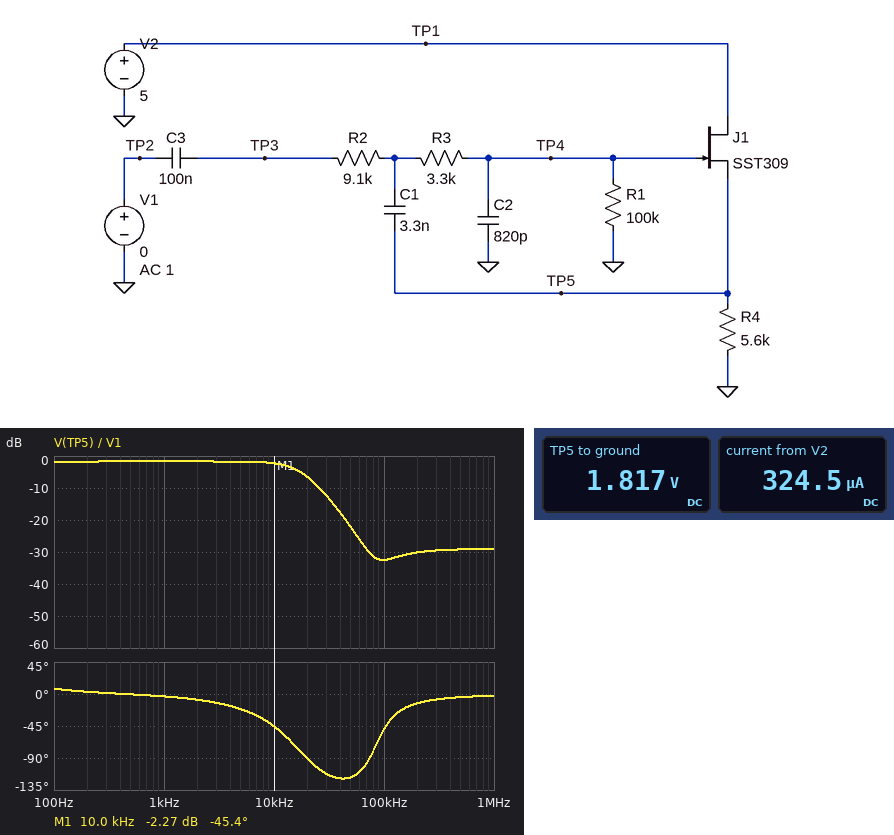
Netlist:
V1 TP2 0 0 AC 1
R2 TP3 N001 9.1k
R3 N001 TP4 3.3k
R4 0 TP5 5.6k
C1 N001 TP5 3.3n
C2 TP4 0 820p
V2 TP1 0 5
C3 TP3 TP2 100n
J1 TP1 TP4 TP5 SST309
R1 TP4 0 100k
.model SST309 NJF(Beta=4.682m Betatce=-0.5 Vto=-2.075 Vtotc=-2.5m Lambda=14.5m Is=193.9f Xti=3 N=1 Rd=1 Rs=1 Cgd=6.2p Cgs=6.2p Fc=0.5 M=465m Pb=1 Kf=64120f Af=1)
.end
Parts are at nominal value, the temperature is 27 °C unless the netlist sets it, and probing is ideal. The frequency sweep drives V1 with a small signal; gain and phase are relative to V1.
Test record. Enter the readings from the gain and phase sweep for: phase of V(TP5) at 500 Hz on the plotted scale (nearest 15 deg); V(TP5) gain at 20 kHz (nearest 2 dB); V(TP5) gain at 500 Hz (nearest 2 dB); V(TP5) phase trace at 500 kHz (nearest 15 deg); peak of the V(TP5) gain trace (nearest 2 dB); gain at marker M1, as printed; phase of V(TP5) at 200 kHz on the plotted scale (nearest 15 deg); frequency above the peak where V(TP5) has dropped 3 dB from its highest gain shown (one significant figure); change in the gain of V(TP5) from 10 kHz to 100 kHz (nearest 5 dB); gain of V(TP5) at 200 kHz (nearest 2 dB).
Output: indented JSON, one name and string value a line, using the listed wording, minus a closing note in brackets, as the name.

{
  "phase of V(TP5) at 500 Hz on the plotted scale": "0 deg",
  "V(TP5) gain at 20 kHz": "-6 dB",
  "V(TP5) gain at 500 Hz": "-2 dB",
  "V(TP5) phase trace at 500 kHz": "0 deg",
  "peak of the V(TP5) gain trace": "-2 dB",
  "gain at marker M1, as printed": "-2.27 dB",
  "phase of V(TP5) at 200 kHz on the plotted scale": "-15 deg",
  "frequency above the peak where V(TP5) has dropped 3 dB from its highest gain shown": "20 kHz",
  "change in the gain of V(TP5) from 10 kHz to 100 kHz": "-30 dB",
  "gain of V(TP5) at 200 kHz": "-30 dB"
}
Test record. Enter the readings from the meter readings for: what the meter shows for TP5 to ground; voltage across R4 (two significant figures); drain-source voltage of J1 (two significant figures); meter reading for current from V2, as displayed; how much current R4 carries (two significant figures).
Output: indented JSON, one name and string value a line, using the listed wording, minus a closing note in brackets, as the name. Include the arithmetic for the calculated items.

{
  "what the meter shows for TP5 to ground": "1.817 V",
  "voltage across R4": "1.817 V = 1.8 V",
  "drain-source voltage of J1": "5 V - 1.817 V = 3.2 V",
  "meter reading for current from V2, as displayed": "324.5 µA",
  "how much current R4 carries": "(1.817 V) / 5.6 kΩ = 320 µA"
}
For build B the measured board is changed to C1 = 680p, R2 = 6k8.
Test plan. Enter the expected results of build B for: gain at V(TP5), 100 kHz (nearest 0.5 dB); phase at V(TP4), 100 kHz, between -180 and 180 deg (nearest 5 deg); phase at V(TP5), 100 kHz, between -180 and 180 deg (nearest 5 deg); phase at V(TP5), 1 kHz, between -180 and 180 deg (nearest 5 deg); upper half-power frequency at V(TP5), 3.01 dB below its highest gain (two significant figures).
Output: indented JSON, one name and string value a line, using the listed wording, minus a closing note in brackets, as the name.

{
  "gain at V(TP5), 100 kHz": "-20.5 dB",
  "phase at V(TP4), 100 kHz, between -180 and 180 deg": "-120 deg",
  "phase at V(TP5), 100 kHz, between -180 and 180 deg": "-115 deg",
  "phase at V(TP5), 1 kHz, between -180 and 180 deg": "0 deg",
  "upper half-power frequency at V(TP5), 3.01 dB below its highest gain": "23 kHz"
}
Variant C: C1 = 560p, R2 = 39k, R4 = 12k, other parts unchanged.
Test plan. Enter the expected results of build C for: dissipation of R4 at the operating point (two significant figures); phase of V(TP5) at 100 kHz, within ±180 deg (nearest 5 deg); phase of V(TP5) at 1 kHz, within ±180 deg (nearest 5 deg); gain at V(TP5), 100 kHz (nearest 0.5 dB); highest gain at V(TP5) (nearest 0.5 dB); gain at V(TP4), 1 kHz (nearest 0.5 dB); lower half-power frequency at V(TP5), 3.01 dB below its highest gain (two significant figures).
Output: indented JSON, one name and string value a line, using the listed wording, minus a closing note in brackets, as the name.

{
  "dissipation of R4 at the operating point": "300 µW",
  "phase of V(TP5) at 100 kHz, within ±180 deg": "-120 deg",
  "phase of V(TP5) at 1 kHz, within ±180 deg": "-10 deg",
  "gain at V(TP5), 100 kHz": "-34.5 dB",
  "highest gain at V(TP5)": "-3.5 dB",
  "gain at V(TP4), 1 kHz": "-3.0 dB",
  "lower half-power frequency at V(TP5), 3.01 dB below its highest gain": "11 Hz"
}
